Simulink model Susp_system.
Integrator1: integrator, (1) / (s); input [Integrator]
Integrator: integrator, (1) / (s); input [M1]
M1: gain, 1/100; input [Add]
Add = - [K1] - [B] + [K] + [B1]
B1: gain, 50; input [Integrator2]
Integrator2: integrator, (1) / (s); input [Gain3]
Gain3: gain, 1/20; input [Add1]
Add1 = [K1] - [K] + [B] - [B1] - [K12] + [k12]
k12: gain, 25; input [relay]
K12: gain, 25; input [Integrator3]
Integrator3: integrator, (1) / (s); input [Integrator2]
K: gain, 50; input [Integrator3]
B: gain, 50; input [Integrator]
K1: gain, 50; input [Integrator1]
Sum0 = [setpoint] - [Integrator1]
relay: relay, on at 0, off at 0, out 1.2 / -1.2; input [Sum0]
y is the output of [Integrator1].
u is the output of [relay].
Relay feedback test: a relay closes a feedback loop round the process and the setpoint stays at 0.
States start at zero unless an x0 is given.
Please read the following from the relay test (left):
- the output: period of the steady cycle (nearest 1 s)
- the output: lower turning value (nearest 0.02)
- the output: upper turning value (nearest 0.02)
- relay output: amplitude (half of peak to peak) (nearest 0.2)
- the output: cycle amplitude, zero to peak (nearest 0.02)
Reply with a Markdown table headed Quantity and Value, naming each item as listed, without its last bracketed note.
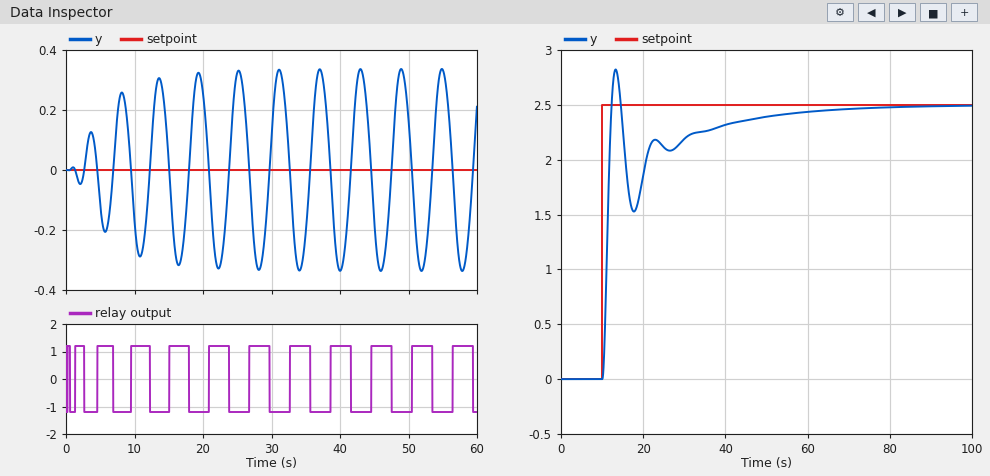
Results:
| Quantity | Value |
|---|---|
| the output: period of the steady cycle | 6 s |
| the output: lower turning value | -0.34 |
| the output: upper turning value | 0.34 |
| relay output: amplitude (half of peak to peak) | 1.2 |
| the output: cycle amplitude, zero to peak | 0.34 |
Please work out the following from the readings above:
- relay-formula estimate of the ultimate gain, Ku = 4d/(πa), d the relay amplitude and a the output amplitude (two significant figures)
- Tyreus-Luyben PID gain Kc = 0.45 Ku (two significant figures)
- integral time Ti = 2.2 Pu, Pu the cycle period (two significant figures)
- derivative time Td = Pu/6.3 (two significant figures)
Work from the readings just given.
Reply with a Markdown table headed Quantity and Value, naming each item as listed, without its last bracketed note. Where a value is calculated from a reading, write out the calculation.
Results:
| Quantity | Value |
|---|---|
| relay-formula estimate of the ultimate gain, Ku = 4d/(πa), d the relay amplitude and a the output amplitude | 4 × 1.2 / (π × 0.34) = 4.5 |
| Tyreus-Luyben PID gain Kc = 0.45 Ku | 0.45 × 4.5 = 2.0 |
| integral time Ti = 2.2 Pu, Pu the cycle period | 2.2 × 6 = 13 s |
| derivative time Td = Pu/6.3 | 6 / 6.3 = 0.95 s |
